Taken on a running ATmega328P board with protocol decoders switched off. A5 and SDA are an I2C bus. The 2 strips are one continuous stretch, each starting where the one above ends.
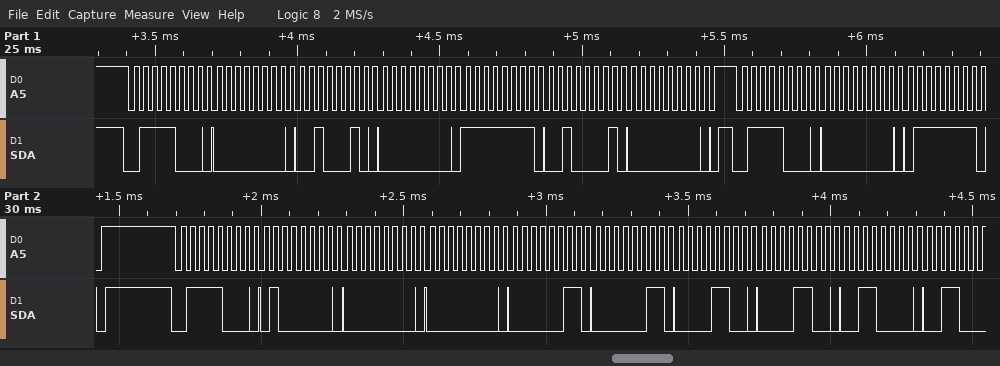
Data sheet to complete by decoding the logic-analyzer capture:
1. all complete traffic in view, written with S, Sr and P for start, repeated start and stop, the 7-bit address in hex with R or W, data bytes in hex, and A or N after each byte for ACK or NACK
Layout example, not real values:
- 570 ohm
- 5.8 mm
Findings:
- S 3CW A 00 A 22 A 00 A FF A 21 A 00 A P S 3CW A 00 A 7F A P S 3CW A 40 A 00 A 00 A 03 A 03 A 0C A 0C A 30 A
